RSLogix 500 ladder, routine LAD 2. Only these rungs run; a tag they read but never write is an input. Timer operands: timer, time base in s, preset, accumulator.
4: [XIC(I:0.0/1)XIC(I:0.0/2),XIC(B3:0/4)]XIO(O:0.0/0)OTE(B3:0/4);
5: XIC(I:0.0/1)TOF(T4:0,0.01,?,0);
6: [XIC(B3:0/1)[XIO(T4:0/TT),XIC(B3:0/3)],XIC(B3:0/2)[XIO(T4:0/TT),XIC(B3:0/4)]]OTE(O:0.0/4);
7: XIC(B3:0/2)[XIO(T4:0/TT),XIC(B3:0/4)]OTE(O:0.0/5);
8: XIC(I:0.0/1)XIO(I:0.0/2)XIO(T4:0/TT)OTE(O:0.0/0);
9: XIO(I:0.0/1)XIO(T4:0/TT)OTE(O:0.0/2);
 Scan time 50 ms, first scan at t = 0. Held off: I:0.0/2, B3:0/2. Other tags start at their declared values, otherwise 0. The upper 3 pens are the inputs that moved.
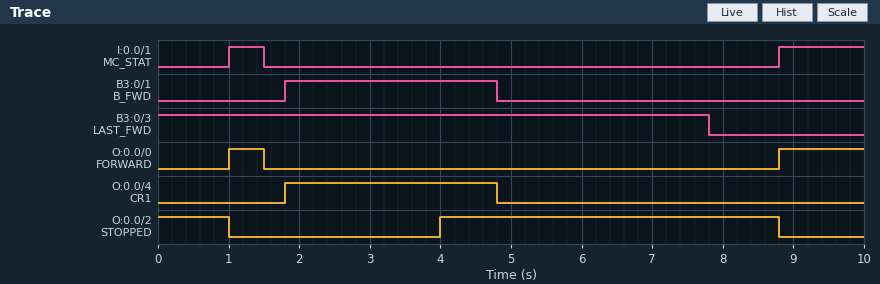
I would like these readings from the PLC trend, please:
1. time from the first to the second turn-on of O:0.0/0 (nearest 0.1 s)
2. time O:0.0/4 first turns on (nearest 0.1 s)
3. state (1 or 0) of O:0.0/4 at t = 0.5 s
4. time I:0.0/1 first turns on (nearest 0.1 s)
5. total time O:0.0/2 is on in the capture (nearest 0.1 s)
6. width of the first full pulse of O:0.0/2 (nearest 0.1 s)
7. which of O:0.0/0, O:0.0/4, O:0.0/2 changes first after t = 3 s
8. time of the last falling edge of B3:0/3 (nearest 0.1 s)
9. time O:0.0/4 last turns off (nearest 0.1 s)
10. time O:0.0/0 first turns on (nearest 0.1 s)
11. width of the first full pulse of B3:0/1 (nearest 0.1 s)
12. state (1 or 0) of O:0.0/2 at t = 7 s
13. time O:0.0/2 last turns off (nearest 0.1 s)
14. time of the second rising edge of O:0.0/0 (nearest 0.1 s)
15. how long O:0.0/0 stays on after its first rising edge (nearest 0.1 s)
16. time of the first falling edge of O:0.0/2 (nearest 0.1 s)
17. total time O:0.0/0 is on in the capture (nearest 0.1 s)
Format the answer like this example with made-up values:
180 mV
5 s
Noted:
7.8 s
1.8 s
0
1.0 s
5.8 s
4.8 s
O:0.0/2
7.8 s
4.8 s
1.0 s
3.0 s
1
8.8 s
8.8 s
0.5 s
1.0 s
1.7 s
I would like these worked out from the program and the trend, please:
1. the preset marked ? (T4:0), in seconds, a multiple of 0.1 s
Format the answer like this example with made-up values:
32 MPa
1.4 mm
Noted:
2.5 s
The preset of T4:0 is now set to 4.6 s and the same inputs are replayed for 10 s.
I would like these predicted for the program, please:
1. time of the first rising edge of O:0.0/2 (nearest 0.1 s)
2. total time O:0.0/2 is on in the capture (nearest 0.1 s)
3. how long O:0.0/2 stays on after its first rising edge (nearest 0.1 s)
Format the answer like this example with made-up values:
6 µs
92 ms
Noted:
6.1 s
3.7 s
2.7 s
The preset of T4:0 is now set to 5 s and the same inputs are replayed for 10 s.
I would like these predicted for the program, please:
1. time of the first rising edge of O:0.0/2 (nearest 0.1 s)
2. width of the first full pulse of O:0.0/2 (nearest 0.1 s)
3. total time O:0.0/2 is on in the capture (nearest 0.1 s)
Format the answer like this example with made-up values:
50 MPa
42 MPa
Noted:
6.5 s
2.3 s
3.3 s
